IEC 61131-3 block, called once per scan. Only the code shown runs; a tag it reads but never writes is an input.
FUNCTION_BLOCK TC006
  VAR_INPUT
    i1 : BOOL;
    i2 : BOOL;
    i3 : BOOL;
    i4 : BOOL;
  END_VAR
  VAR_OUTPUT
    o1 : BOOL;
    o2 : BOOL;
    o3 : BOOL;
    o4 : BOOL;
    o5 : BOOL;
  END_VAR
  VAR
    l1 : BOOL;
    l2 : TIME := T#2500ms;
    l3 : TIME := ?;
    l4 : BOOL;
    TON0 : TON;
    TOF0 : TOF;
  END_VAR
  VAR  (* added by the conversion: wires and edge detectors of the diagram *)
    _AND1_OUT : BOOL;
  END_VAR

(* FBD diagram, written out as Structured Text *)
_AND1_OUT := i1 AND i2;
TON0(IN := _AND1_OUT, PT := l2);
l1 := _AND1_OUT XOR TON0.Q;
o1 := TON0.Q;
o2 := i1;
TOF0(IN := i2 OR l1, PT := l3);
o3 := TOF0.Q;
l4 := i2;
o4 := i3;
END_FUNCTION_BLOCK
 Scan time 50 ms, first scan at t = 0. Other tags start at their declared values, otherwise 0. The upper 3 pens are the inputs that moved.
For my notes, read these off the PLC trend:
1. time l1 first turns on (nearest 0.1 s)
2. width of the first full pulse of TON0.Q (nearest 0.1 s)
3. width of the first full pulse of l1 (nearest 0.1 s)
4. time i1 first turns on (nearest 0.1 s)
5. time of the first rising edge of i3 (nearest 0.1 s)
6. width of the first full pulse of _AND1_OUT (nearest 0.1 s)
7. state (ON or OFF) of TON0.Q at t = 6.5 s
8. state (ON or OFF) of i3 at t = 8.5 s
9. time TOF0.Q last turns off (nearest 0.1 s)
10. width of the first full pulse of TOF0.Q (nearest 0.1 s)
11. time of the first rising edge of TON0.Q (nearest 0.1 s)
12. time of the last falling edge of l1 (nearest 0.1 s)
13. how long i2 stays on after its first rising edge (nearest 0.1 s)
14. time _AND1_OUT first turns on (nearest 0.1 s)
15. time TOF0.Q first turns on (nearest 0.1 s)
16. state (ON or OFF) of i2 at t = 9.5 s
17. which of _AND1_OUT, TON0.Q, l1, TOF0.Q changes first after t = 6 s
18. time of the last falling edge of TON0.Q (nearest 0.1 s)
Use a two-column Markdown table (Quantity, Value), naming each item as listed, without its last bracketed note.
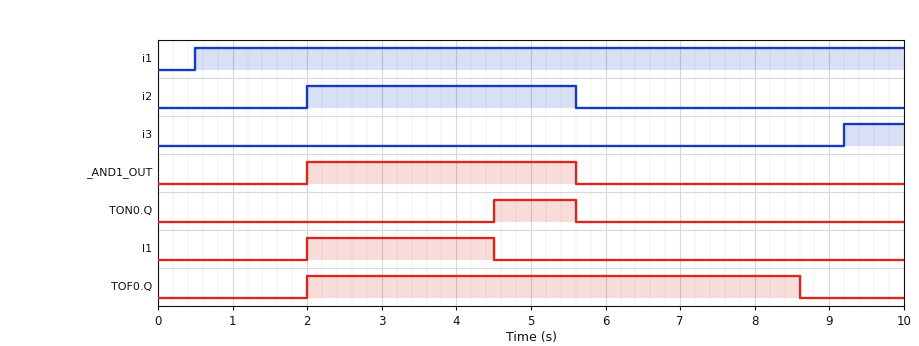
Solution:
| Quantity | Value |
|---|---|
| time l1 first turns on | 2.0 s |
| width of the first full pulse of TON0.Q | 1.1 s |
| width of the first full pulse of l1 | 2.5 s |
| time i1 first turns on | 0.5 s |
| time of the first rising edge of i3 | 9.2 s |
| width of the first full pulse of _AND1_OUT | 3.6 s |
| state (ON or OFF) of TON0.Q at t = 6.5 s | OFF |
| state (ON or OFF) of i3 at t = 8.5 s | OFF |
| time TOF0.Q last turns off | 8.6 s |
| width of the first full pulse of TOF0.Q | 6.6 s |
| time of the first rising edge of TON0.Q | 4.5 s |
| time of the last falling edge of l1 | 4.5 s |
| how long i2 stays on after its first rising edge | 3.6 s |
| time _AND1_OUT first turns on | 2.0 s |
| time TOF0.Q first turns on | 2.0 s |
| state (ON or OFF) of i2 at t = 9.5 s | OFF |
| which of _AND1_OUT, TON0.Q, l1, TOF0.Q changes first after t = 6 s | TOF0.Q |
| time of the last falling edge of TON0.Q | 5.6 s |
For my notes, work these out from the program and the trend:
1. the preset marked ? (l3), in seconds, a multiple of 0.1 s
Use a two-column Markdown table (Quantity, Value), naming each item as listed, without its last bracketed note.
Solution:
| Quantity | Value |
|---|---|
| the preset marked ? (l3), in seconds, a multiple of 0.1 s | 3.0 s |
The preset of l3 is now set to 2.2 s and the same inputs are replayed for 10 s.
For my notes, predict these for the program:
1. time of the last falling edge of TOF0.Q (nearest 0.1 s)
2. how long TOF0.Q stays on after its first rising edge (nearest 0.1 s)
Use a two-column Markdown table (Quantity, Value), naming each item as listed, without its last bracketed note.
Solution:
| Quantity | Value |
|---|---|
| time of the last falling edge of TOF0.Q | 7.8 s |
| how long TOF0.Q stays on after its first rising edge | 5.8 s |
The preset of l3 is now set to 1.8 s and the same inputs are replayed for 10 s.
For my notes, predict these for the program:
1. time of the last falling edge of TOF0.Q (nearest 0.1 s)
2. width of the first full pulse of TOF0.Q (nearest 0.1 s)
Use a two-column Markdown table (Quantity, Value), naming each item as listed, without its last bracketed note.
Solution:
| Quantity | Value |
|---|---|
| time of the last falling edge of TOF0.Q | 7.4 s |
| width of the first full pulse of TOF0.Q | 5.4 s |
